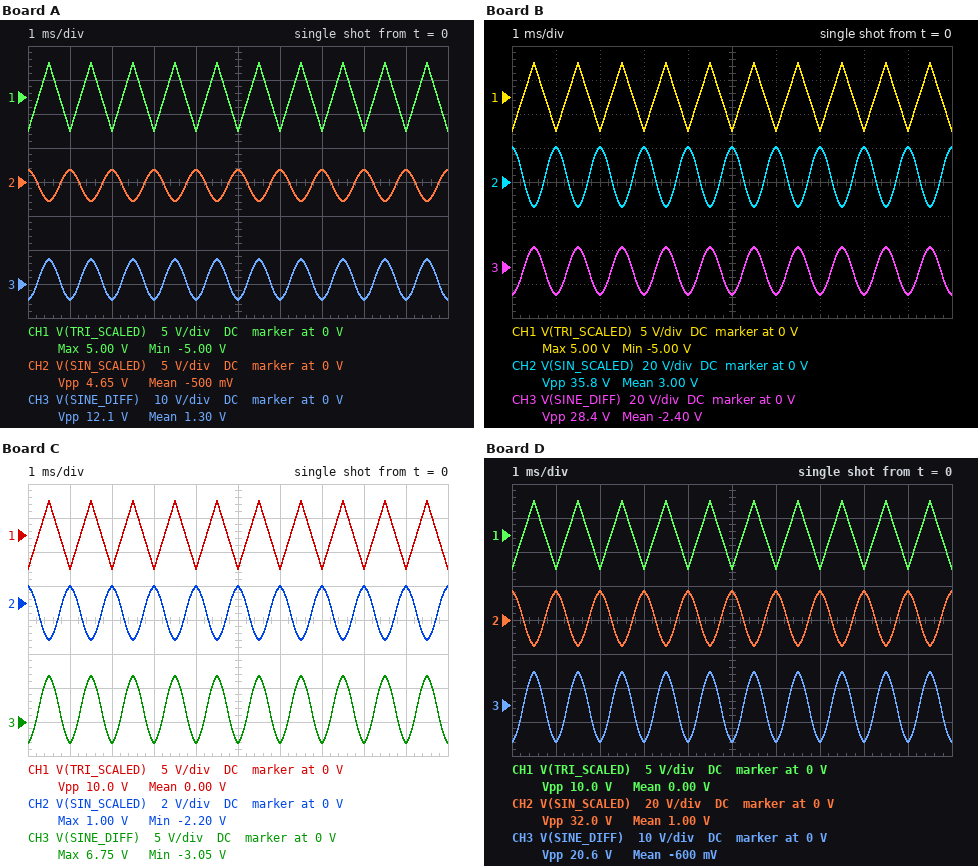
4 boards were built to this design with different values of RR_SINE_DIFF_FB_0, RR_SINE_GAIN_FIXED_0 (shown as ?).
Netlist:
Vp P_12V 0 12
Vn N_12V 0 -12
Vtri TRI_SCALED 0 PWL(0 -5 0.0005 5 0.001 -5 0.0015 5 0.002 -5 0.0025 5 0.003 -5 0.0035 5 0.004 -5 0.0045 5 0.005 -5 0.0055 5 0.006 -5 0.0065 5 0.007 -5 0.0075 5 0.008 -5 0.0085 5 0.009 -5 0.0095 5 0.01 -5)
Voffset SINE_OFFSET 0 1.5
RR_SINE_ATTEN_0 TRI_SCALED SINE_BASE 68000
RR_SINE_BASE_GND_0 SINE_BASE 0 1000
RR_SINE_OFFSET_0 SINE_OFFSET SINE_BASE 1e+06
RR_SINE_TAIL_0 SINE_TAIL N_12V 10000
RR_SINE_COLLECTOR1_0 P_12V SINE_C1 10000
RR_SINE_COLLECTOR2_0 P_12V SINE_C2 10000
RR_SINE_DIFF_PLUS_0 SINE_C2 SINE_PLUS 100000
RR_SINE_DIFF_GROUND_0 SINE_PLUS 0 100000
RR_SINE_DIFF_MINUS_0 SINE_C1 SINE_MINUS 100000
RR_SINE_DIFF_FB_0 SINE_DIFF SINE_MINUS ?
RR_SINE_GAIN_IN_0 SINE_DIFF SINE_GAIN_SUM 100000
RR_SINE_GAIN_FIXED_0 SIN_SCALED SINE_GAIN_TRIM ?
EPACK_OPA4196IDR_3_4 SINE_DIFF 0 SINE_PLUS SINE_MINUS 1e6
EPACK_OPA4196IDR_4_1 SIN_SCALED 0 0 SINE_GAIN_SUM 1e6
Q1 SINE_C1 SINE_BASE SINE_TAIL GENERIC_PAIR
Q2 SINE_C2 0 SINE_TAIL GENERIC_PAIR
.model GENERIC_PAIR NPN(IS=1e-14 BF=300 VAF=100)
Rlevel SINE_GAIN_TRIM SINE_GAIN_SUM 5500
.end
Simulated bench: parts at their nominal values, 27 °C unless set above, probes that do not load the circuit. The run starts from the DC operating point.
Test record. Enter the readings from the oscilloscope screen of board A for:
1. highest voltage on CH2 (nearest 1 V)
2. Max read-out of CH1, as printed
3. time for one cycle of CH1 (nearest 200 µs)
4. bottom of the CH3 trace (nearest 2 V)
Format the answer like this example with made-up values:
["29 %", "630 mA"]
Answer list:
["2 V", "5.00 V", "1.0 ms", "-4 V"]
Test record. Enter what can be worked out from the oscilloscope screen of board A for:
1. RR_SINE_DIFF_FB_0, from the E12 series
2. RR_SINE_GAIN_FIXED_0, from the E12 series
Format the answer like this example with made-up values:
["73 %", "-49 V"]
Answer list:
["56 kΩ", "33 kΩ"]
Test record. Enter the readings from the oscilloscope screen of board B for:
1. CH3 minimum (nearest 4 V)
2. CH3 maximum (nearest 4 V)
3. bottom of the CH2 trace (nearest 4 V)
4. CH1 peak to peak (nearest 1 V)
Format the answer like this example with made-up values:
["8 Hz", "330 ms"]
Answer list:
["-16 V", "12 V", "-16 V", "10 V"]
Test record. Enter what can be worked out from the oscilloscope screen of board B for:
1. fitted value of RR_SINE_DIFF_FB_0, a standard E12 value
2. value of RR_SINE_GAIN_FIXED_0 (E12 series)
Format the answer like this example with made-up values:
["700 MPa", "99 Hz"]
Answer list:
["180 kΩ", "120 kΩ"]
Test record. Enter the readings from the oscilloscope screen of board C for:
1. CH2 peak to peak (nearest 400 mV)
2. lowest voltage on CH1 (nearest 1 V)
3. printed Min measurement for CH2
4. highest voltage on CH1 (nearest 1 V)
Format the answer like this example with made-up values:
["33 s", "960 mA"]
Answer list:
["3.2 V", "-5 V", "-2.20 V", "5 V"]
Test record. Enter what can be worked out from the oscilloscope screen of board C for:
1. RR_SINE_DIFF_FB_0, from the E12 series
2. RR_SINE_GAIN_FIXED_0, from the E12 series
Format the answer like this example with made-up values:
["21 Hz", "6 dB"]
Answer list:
["39 kΩ", "27 kΩ"]
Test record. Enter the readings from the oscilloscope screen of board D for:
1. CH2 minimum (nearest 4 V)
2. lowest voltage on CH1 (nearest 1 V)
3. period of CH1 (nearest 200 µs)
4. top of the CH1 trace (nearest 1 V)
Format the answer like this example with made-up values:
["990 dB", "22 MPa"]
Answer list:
["-16 V", "-5 V", "1.0 ms", "5 V"]
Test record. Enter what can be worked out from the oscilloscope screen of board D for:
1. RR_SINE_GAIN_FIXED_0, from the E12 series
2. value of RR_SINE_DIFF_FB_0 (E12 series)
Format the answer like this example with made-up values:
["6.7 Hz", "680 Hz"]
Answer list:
["150 kΩ", "120 kΩ"]
